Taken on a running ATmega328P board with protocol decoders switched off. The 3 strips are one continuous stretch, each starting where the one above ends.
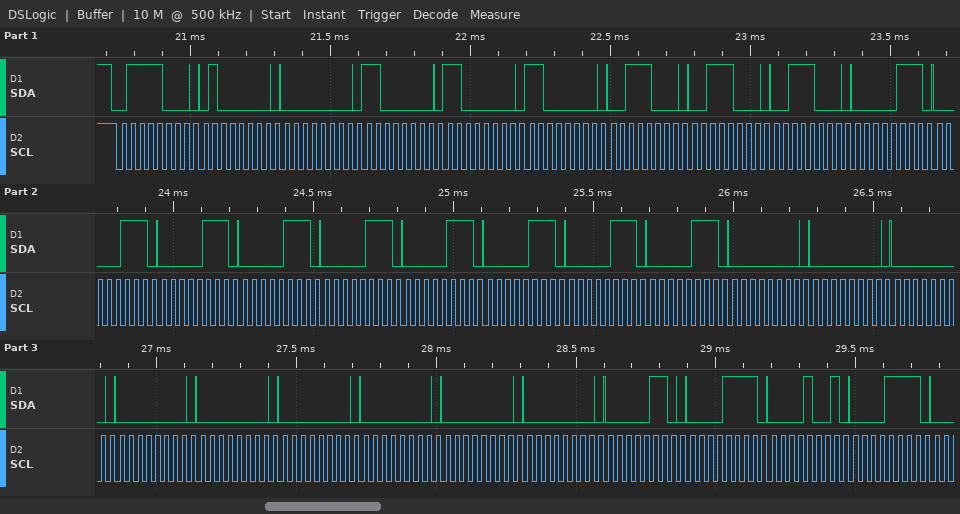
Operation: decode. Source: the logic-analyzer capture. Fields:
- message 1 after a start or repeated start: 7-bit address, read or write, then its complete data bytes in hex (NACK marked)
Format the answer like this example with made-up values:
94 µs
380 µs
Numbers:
0x3C write: 40 00 C0 C0 C0 38 38 38 07 07 07 07 07 07 07 07 07 00 00 00 00 00 00 00 00 00 06 0F 09 0F
